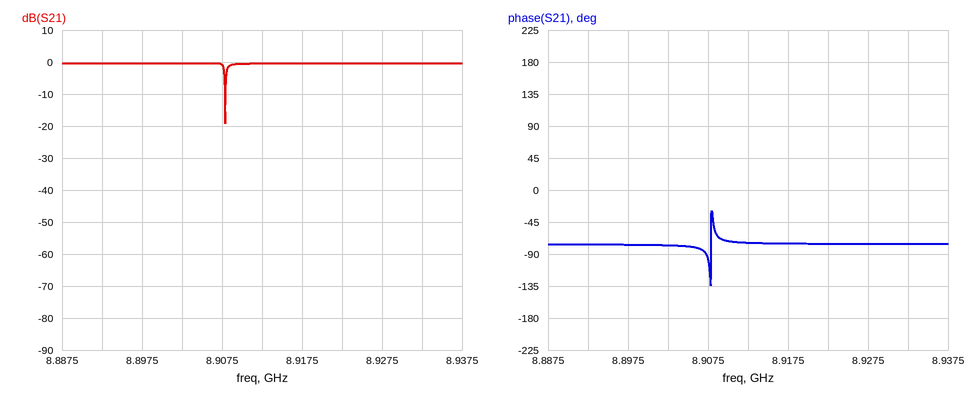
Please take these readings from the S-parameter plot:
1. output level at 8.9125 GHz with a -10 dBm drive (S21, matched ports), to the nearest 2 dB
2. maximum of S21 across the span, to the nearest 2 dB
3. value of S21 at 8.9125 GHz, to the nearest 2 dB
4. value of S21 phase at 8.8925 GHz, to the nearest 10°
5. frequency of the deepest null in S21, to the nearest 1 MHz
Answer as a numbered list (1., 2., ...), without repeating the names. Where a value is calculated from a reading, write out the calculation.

1. -10 dBm + (0 dB) = -10 dBm
2. 0 dB
3. 0 dB
4. -80°
5. 8.908 GHz
